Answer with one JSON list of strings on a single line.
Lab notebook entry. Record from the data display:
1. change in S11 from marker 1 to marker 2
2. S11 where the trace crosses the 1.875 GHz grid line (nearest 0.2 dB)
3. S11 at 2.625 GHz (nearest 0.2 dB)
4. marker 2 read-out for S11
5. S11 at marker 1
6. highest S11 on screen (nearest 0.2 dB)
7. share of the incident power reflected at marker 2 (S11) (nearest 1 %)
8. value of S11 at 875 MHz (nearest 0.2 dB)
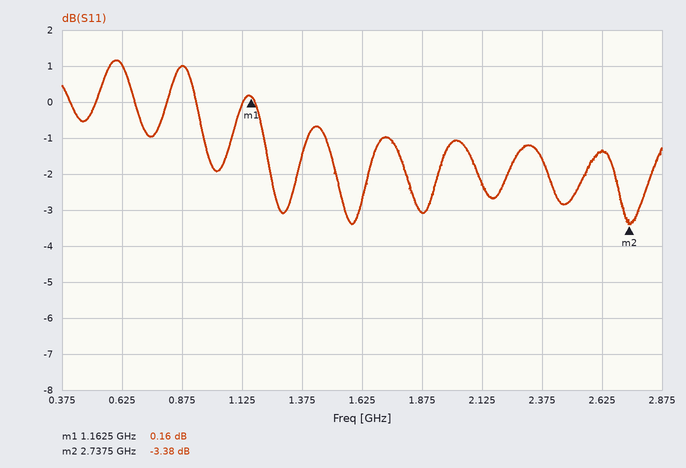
["-3.54 dB", "-3.0 dB", "-1.4 dB", "-3.38 dB", "0.16 dB", "1.2 dB", "46 %", "1.0 dB"]
